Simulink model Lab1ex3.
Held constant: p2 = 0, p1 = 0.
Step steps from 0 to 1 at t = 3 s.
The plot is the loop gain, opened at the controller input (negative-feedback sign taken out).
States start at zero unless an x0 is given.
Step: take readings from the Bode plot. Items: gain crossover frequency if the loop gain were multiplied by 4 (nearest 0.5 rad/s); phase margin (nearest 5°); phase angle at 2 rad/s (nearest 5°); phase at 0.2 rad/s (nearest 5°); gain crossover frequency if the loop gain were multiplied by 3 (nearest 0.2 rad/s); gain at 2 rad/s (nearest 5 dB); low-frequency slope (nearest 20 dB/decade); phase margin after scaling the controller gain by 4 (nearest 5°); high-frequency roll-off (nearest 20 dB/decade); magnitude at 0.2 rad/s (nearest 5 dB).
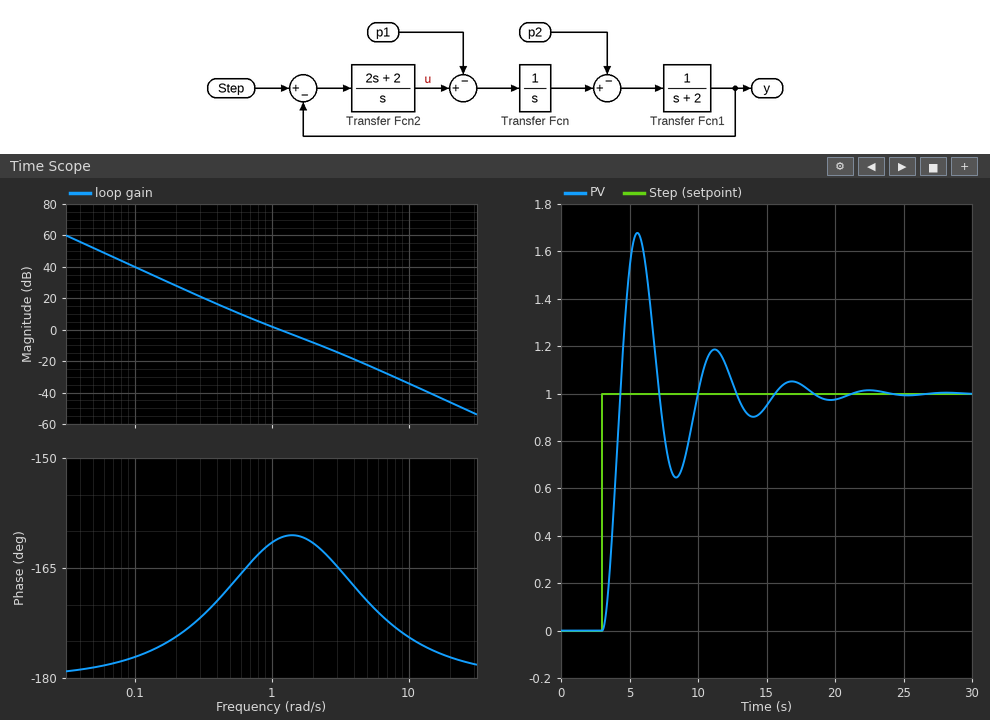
2.5 rad/s
20°
-160°
-175°
2.2 rad/s
-10 dB
-40 dB/decade
15°
-40 dB/decade
30 dB
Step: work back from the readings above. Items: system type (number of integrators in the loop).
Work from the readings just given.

2
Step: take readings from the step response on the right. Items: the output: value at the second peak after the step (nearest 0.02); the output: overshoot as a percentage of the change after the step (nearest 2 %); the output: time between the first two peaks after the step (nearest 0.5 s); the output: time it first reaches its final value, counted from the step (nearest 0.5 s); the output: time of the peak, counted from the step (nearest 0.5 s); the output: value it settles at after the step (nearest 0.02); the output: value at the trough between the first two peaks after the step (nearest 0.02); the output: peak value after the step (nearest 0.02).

1.18
68 %
5.5 s
1.5 s
2.5 s
1.00
0.64
1.68
